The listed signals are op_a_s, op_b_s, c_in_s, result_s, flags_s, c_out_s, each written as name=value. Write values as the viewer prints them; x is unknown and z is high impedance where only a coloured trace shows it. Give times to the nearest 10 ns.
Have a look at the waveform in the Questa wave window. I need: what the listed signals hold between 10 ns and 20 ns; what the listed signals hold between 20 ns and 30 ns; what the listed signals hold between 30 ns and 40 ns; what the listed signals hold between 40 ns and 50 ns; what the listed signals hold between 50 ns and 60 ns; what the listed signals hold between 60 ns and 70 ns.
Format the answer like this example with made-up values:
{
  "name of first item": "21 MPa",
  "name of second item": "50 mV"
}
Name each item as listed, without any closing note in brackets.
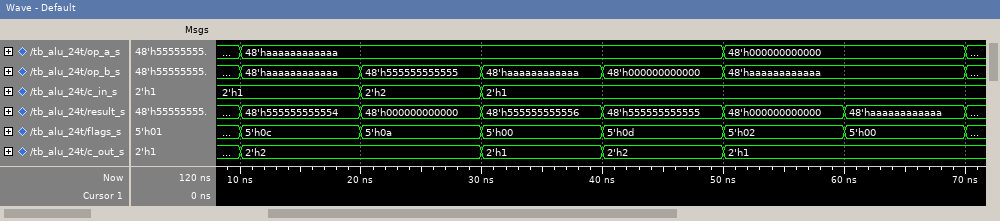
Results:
{
  "what the listed signals hold between 10 ns and 20 ns": "op_a_s=48'haaaaaaaaaaaa, op_b_s=48'haaaaaaaaaaaa, c_in_s=2'h1, result_s=48'h555555555554, flags_s=5'h0c, c_out_s=2'h2",
  "what the listed signals hold between 20 ns and 30 ns": "op_a_s=48'haaaaaaaaaaaa, op_b_s=48'h555555555555, c_in_s=2'h2, result_s=48'h000000000000, flags_s=5'h0a, c_out_s=2'h2",
  "what the listed signals hold between 30 ns and 40 ns": "op_a_s=48'haaaaaaaaaaaa, op_b_s=48'haaaaaaaaaaaa, c_in_s=2'h1, result_s=48'h555555555556, flags_s=5'h00, c_out_s=2'h1",
  "what the listed signals hold between 40 ns and 50 ns": "op_a_s=48'haaaaaaaaaaaa, op_b_s=48'h000000000000, c_in_s=2'h1, result_s=48'h555555555555, flags_s=5'h0d, c_out_s=2'h2",
  "what the listed signals hold between 50 ns and 60 ns": "op_a_s=48'h000000000000, op_b_s=48'haaaaaaaaaaaa, c_in_s=2'h1, result_s=48'h000000000000, flags_s=5'h02, c_out_s=2'h1",
  "what the listed signals hold between 60 ns and 70 ns": "op_a_s=48'h000000000000, op_b_s=48'haaaaaaaaaaaa, c_in_s=2'h1, result_s=48'haaaaaaaaaaaa, flags_s=5'h00, c_out_s=2'h1"
}
